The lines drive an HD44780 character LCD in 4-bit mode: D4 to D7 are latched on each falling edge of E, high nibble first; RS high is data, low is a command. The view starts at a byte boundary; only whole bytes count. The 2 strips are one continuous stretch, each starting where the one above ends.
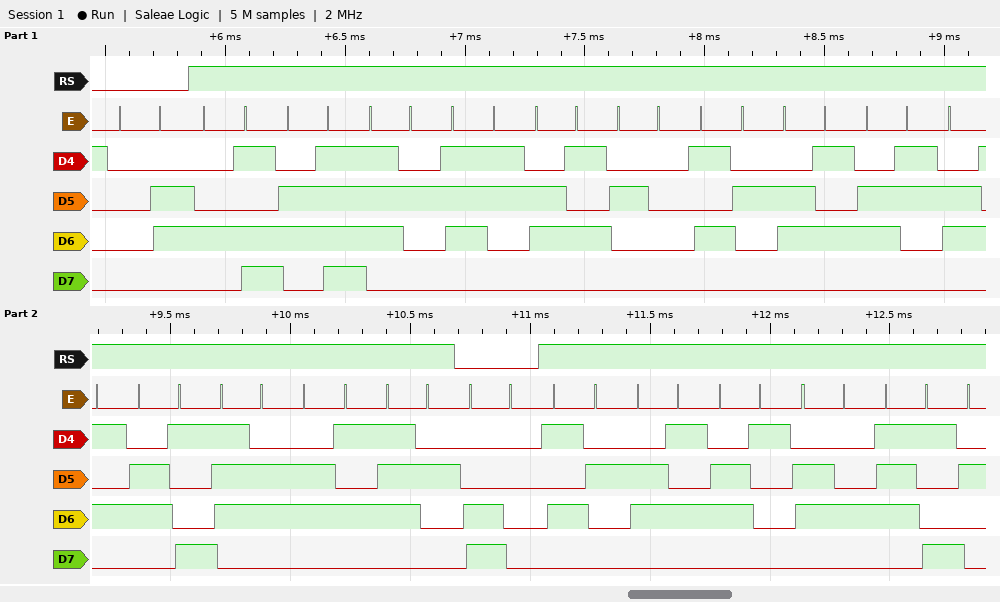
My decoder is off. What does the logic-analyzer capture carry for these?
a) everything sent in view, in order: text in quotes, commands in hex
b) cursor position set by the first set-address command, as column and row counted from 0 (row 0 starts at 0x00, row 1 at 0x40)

0x06 "Morse Receiver" 0xC0 "Ready"
column 0, row 1
